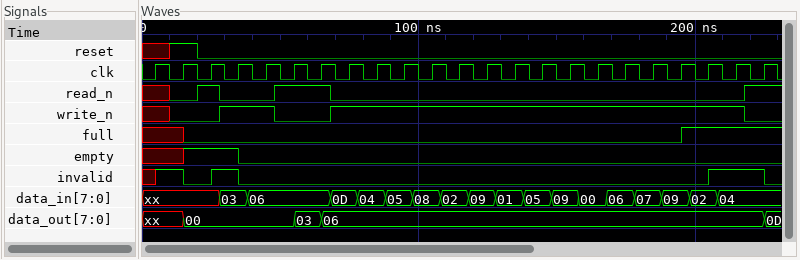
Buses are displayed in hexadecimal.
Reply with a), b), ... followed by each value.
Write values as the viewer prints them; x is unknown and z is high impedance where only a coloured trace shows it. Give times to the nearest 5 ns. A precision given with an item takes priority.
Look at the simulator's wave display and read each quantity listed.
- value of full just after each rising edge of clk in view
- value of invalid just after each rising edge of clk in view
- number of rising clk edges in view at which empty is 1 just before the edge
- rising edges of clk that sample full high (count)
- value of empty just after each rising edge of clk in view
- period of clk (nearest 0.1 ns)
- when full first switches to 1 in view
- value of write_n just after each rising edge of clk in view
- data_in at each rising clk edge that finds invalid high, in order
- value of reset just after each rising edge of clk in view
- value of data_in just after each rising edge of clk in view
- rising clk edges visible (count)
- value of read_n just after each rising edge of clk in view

a) x 0 0 0 0 0 0 0 0 0 0 0 0 0 0 0 0 0 0 1 1 1 1
b) 1 0 1 0 0 0 0 0 0 0 0 0 0 0 0 0 0 0 0 0 1 1 0
c) 2
d) 3
e) x 1 1 0 0 0 0 0 0 0 0 0 0 0 0 0 0 0 0 0 0 0 0
f) 10 ns
g) 195 ns
h) x 0 0 1 1 0 0 1 1 1 1 1 1 1 1 1 1 1 1 1 1 1 0
i) xx, 03, 04, 04
j) x 1 0 0 0 0 0 0 0 0 0 0 0 0 0 0 0 0 0 0 0 0 0
k) xx, xx, xx, 03, 06, 06, 06, 0D, 04, 05, 08, 02, 09, 01, 05, 09, 00, 06, 07, 09, 02, 04, 04
l) 23
m) x 0 1 0 0 1 1 0 0 0 0 0 0 0 0 0 0 0 0 0 0 0 1
